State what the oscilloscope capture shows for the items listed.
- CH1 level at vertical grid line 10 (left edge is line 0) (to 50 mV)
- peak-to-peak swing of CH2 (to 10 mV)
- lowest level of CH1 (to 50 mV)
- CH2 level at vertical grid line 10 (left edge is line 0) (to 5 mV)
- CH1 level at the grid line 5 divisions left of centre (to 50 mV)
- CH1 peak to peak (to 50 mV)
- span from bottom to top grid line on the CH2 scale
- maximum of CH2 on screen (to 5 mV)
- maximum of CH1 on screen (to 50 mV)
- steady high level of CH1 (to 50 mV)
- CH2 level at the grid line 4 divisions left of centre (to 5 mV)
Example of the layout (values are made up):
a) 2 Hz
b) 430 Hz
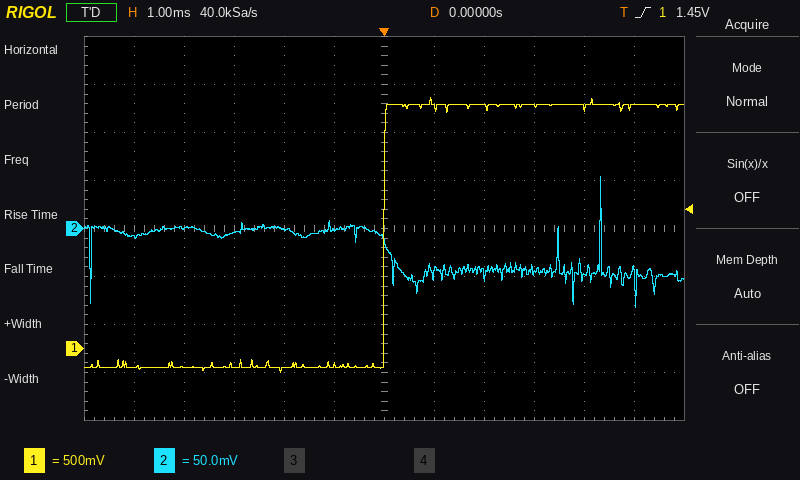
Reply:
a) 2.50 V
b) 140 mV
c) -250 mV
d) -50 mV
e) -200 mV
f) 2.85 V
g) 400 mV
h) 55 mV
i) 2.60 V
j) 2.55 V
k) 0 mV
